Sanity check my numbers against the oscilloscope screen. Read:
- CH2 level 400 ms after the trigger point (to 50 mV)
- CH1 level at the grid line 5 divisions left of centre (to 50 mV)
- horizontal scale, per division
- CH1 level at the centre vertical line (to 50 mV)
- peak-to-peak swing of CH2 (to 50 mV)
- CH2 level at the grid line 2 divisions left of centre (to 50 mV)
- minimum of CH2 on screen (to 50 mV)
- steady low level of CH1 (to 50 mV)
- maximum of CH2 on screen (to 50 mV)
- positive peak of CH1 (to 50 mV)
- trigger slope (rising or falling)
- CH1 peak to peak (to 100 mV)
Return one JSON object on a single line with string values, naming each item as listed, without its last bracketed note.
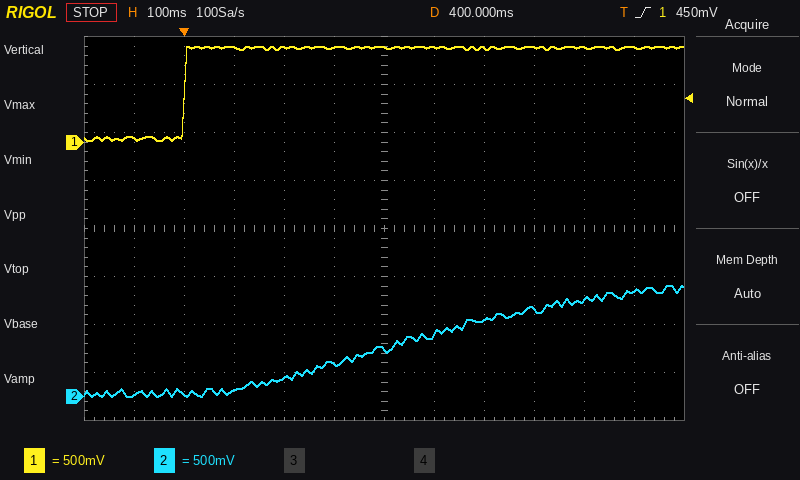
{"CH2 level 400 ms after the trigger point": "500 mV", "CH1 level at the grid line 5 divisions left of centre": "50 mV", "horizontal scale, per division": "100 ms", "CH1 level at the centre vertical line": "1.00 V", "peak-to-peak swing of CH2": "1.15 V", "CH2 level at the grid line 2 divisions left of centre": "200 mV", "minimum of CH2 on screen": "0 mV", "steady low level of CH1": "50 mV", "maximum of CH2 on screen": "1.15 V", "positive peak of CH1": "1.00 V", "trigger slope": "rising", "CH1 peak to peak": "1.00 V"}
